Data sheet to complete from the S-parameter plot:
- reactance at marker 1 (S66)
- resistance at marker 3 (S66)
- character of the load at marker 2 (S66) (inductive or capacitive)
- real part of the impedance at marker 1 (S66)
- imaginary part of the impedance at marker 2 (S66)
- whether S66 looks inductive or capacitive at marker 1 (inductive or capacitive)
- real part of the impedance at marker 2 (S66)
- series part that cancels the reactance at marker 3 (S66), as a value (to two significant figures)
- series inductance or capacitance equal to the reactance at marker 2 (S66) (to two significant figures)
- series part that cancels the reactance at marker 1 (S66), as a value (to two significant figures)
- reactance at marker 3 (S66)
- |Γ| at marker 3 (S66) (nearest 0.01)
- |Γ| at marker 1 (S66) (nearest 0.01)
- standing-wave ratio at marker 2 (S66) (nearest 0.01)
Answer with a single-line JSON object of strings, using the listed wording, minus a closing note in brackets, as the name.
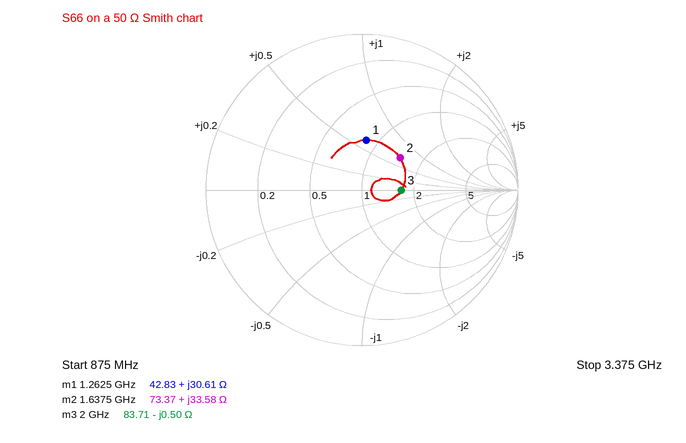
{"reactance at marker 1": "+30.61 Ω", "resistance at marker 3": "83.71 Ω", "character of the load at marker 2 (S66)": "inductive", "real part of the impedance at marker 1": "42.83 Ω", "imaginary part of the impedance at marker 2": "+33.58 Ω", "whether S66 looks inductive or capacitive at marker 1": "inductive", "real part of the impedance at marker 2": "73.37 Ω", "series part that cancels the reactance at marker 3 (S66), as a value": "40 pH", "series inductance or capacitance equal to the reactance at marker 2 (S66)": "3.3 nH", "series part that cancels the reactance at marker 1 (S66), as a value": "4.1 pF", "reactance at marker 3": "-0.50 Ω", "|Γ| at marker 3 (S66)": "0.25", "|Γ| at marker 1 (S66)": "0.32", "standing-wave ratio at marker 2 (S66)": "1.94"}
